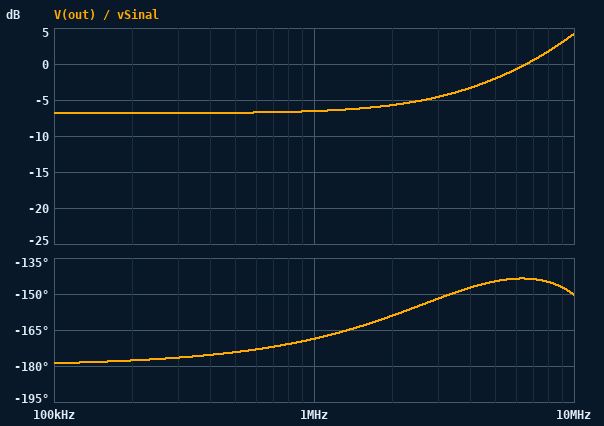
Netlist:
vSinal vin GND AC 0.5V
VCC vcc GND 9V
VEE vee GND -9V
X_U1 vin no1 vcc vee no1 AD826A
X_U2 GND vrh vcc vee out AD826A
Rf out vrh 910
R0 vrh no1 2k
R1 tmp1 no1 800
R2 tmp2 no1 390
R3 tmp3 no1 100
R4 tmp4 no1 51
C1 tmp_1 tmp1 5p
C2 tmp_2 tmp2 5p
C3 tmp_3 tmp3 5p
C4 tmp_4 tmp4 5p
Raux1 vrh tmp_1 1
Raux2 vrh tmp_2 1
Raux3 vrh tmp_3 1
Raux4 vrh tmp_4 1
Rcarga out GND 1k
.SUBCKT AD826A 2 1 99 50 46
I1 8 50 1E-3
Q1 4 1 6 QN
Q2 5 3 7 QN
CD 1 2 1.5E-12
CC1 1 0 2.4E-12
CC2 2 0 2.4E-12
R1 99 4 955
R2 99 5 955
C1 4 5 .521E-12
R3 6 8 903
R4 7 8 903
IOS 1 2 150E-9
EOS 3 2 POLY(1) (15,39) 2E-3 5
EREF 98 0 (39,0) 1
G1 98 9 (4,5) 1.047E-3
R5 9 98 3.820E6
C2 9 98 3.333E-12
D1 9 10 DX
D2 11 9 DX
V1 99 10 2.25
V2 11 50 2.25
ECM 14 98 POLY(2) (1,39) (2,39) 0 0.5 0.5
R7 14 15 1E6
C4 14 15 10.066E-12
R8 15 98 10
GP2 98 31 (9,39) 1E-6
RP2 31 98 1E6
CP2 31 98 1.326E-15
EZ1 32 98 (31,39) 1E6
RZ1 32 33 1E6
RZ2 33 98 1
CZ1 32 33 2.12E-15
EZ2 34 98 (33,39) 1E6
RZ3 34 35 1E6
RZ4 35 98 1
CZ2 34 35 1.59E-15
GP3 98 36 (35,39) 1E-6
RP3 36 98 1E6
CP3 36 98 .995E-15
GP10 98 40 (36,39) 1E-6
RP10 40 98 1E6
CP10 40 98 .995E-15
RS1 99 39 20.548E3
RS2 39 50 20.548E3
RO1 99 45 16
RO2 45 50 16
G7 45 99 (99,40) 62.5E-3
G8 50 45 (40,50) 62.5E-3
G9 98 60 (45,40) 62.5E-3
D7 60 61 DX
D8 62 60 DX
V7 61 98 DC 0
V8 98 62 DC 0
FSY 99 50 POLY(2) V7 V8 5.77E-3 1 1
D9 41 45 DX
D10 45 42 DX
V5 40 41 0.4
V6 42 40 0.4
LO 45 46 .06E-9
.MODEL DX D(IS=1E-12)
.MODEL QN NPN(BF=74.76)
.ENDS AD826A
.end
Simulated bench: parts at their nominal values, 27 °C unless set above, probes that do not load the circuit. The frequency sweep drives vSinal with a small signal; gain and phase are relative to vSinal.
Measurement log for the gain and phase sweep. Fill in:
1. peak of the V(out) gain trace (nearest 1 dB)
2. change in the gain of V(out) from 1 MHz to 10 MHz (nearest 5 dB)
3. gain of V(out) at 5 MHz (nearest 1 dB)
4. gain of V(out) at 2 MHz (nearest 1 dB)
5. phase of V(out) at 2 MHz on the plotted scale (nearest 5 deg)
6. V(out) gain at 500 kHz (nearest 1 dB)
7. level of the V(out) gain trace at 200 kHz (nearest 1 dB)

4 dB
10 dB
-2 dB
-6 dB
-160 deg
-7 dB
-7 dB
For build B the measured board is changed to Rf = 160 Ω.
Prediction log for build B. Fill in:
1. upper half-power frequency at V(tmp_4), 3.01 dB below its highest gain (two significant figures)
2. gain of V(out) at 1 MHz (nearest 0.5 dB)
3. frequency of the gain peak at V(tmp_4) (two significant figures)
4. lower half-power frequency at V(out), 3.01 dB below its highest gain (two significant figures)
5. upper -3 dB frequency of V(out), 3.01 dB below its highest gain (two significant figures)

110 MHz
-21.5 dB
56 MHz
25 MHz
69 MHz
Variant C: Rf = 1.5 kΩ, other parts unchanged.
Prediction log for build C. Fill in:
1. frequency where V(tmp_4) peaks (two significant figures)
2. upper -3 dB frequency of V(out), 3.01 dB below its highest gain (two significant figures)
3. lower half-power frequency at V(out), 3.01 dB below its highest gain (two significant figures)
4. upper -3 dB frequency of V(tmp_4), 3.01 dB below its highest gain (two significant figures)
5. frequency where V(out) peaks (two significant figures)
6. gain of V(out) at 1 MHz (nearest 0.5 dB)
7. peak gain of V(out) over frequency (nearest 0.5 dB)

16 MHz
19 MHz
11 MHz
25 MHz
14 MHz
-2.0 dB
14.0 dB
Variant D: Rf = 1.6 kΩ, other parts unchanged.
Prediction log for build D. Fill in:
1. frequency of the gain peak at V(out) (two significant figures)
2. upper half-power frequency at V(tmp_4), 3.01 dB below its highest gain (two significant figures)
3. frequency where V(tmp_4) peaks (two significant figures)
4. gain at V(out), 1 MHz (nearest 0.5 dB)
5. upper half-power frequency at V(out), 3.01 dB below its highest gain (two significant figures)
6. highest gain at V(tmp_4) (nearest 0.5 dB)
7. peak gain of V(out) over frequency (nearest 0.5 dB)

14 MHz
24 MHz
15 MHz
-1.5 dB
18 MHz
4.0 dB
14.5 dB
